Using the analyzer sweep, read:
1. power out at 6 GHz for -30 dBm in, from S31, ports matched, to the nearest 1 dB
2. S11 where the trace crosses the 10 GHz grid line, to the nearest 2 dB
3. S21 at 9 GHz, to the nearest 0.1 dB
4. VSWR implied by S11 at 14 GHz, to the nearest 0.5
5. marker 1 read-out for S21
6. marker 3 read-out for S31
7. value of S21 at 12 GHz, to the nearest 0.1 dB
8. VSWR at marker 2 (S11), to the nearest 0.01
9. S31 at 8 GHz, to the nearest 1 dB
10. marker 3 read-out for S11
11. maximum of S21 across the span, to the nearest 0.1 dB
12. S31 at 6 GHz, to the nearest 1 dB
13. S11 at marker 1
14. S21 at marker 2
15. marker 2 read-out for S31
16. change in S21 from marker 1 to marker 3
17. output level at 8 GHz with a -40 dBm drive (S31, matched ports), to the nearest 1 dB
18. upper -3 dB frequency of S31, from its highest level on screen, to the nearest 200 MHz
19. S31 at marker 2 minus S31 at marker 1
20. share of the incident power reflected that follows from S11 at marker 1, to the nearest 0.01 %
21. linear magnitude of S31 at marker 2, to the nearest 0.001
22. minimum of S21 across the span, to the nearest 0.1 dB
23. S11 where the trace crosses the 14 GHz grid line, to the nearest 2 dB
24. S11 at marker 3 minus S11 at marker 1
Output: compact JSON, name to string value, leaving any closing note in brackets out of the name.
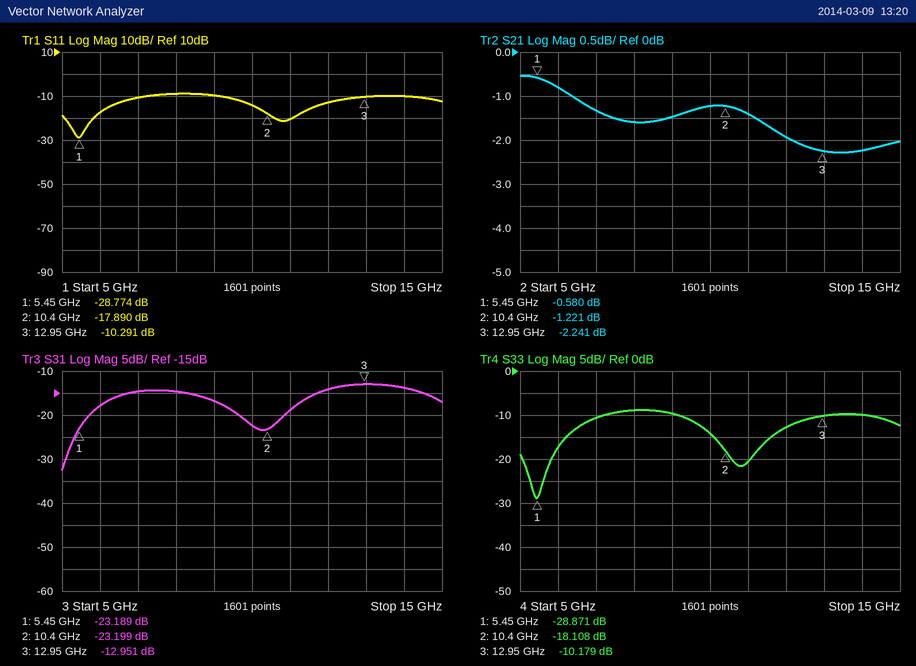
{"power out at 6 GHz for -30 dBm in, from S31, ports matched, to the nearest 1 dB": "-48 dBm", "S11 where the trace crosses the 10 GHz grid line, to the nearest 2 dB": "-14 dB", "S21 at 9 GHz, to the nearest 0.1 dB": "-1.5 dB", "VSWR implied by S11 at 14 GHz, to the nearest 0.5": "2.0", "marker 1 read-out for S21": "-0.580 dB", "marker 3 read-out for S31": "-12.951 dB", "value of S21 at 12 GHz, to the nearest 0.1 dB": "-1.9 dB", "VSWR at marker 2 (S11), to the nearest 0.01": "1.29", "S31 at 8 GHz, to the nearest 1 dB": "-15 dB", "marker 3 read-out for S11": "-10.291 dB", "maximum of S21 across the span, to the nearest 0.1 dB": "-0.5 dB", "S31 at 6 GHz, to the nearest 1 dB": "-18 dB", "S11 at marker 1": "-28.774 dB", "S21 at marker 2": "-1.221 dB", "marker 2 read-out for S31": "-23.199 dB", "change in S21 from marker 1 to marker 3": "-1.661 dB", "output level at 8 GHz with a -40 dBm drive (S31, matched ports), to the nearest 1 dB": "-55 dBm", "upper -3 dB frequency of S31, from its highest level on screen, to the nearest 200 MHz": "14.8 GHz", "S31 at marker 2 minus S31 at marker 1": "-0.010 dB", "share of the incident power reflected that follows from S11 at marker 1, to the nearest 0.01 %": "0.13 %", "linear magnitude of S31 at marker 2, to the nearest 0.001": "0.069", "minimum of S21 across the span, to the nearest 0.1 dB": "-2.3 dB", "S11 where the trace crosses the 14 GHz grid line, to the nearest 2 dB": "-10 dB", "S11 at marker 3 minus S11 at marker 1": "18.483 dB"}
